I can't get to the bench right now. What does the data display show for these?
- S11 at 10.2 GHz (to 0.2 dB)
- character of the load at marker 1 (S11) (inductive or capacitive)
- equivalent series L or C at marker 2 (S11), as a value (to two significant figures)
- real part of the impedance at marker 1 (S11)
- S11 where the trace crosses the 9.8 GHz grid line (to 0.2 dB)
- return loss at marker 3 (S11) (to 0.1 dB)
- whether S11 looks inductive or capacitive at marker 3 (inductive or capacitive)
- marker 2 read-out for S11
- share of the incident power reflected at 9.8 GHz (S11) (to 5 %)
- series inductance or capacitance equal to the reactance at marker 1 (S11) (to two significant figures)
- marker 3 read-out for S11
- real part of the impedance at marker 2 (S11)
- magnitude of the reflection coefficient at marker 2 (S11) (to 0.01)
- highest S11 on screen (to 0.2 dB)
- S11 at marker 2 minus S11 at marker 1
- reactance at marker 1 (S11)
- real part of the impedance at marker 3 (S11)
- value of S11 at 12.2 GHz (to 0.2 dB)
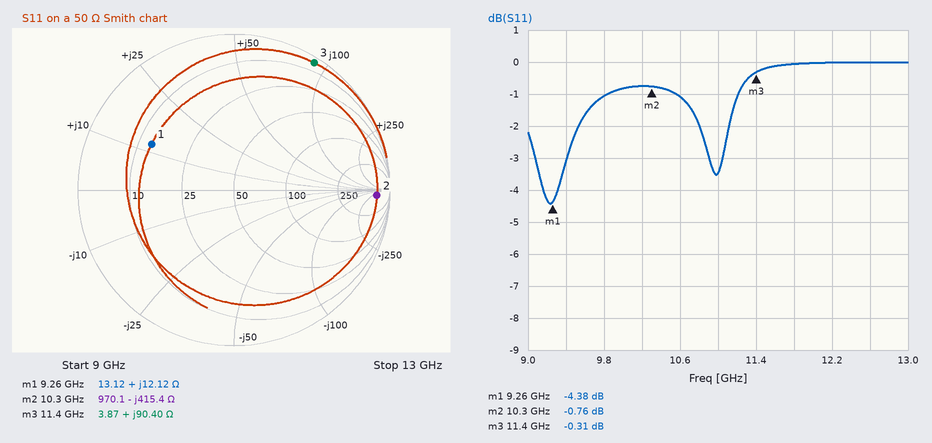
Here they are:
-0.8 dB
inductive
37 fF
13.12 Ω
-1.0 dB
0.3 dB
inductive
-0.76 dB
80 %
210 pH
-0.31 dB
970.1 Ω
0.92
0.0 dB
3.62 dB
+12.12 Ω
3.87 Ω
0.0 dB
